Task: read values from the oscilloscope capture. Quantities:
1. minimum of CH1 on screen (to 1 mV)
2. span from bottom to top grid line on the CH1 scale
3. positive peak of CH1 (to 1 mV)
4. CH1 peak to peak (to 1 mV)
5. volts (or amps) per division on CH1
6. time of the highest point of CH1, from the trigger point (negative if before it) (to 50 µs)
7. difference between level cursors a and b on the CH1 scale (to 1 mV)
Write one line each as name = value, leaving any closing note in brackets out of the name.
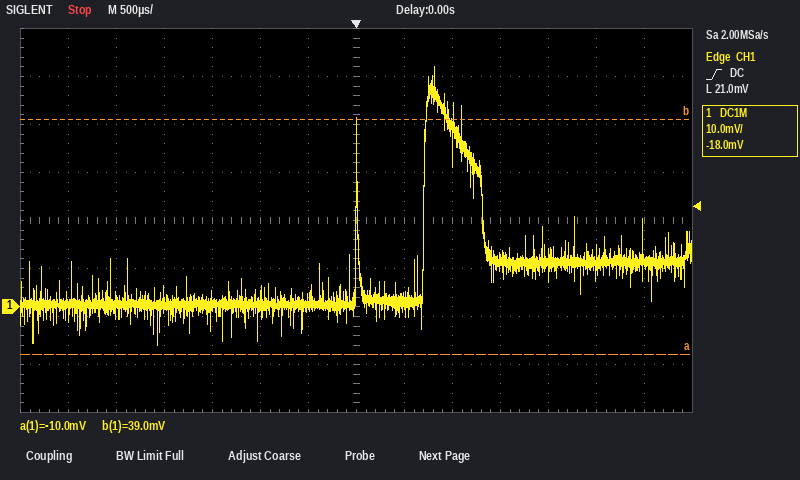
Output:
minimum of CH1 on screen = -8 mV
span from bottom to top grid line on the CH1 scale = 80 mV
positive peak of CH1 = 50 mV
CH1 peak to peak = 58 mV
volts (or amps) per division on CH1 = 10 mV
time of the highest point of CH1, from the trigger point (negative if before it) = +800 µs
difference between level cursors a and b on the CH1 scale = 49 mV
